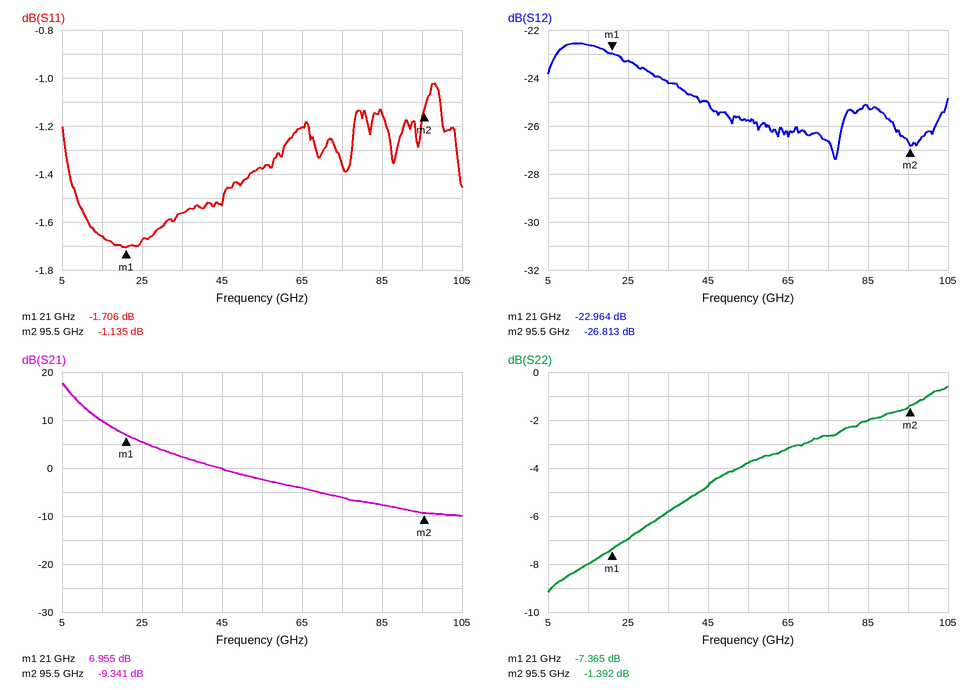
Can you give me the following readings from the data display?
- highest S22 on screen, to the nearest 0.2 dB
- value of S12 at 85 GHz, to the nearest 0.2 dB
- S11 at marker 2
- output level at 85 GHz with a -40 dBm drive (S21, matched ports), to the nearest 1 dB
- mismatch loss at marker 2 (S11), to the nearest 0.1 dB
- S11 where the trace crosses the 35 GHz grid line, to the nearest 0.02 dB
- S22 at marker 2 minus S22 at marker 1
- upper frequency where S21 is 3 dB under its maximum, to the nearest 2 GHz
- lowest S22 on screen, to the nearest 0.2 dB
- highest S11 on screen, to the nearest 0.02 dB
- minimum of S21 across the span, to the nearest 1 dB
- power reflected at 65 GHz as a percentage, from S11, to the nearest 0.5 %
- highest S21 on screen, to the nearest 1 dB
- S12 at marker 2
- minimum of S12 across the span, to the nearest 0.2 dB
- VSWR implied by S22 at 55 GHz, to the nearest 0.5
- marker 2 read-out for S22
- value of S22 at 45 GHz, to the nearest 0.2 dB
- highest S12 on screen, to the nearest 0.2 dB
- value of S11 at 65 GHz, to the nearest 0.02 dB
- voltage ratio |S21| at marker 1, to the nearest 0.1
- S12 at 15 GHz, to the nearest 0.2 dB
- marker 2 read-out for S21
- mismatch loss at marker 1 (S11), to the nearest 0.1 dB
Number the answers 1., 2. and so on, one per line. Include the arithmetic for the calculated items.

1. -0.6 dB
2. -25.2 dB
3. -1.135 dB
4. -40 dBm + (-8 dB) = -48 dBm
5. −10 log10(1 − 10^(-1.135/10)) ≈ 6.4 dB
6. -1.56 dB
7. -1.392 − (-7.365) = 5.973 dB
8. 8 GHz
9. -9.2 dB
10. -1.02 dB
11. -10 dB
12. 10^(-1.2/10) ≈ 75.9 %, so 76.0 % to the nearest 0.5 %
13. 18 dB
14. -26.813 dB
15. -27.4 dB
16. |Γ| = 10^(-3.8/20) = 0.6457; VSWR = (1 + 0.6457)/(1 − 0.6457) ≈ 4.64, so 4.5 to the nearest 0.5
17. -1.392 dB
18. -4.8 dB
19. -22.6 dB
20. -1.20 dB
21. 10^(6.955/20) ≈ 2.2
22. -22.6 dB
23. -9.341 dB
24. −10 log10(1 − 10^(-1.706/10)) ≈ 4.9 dB
